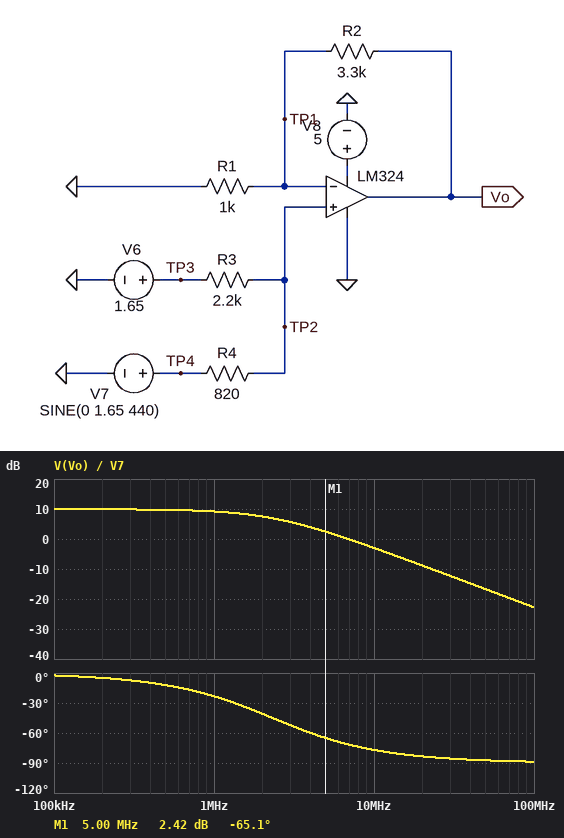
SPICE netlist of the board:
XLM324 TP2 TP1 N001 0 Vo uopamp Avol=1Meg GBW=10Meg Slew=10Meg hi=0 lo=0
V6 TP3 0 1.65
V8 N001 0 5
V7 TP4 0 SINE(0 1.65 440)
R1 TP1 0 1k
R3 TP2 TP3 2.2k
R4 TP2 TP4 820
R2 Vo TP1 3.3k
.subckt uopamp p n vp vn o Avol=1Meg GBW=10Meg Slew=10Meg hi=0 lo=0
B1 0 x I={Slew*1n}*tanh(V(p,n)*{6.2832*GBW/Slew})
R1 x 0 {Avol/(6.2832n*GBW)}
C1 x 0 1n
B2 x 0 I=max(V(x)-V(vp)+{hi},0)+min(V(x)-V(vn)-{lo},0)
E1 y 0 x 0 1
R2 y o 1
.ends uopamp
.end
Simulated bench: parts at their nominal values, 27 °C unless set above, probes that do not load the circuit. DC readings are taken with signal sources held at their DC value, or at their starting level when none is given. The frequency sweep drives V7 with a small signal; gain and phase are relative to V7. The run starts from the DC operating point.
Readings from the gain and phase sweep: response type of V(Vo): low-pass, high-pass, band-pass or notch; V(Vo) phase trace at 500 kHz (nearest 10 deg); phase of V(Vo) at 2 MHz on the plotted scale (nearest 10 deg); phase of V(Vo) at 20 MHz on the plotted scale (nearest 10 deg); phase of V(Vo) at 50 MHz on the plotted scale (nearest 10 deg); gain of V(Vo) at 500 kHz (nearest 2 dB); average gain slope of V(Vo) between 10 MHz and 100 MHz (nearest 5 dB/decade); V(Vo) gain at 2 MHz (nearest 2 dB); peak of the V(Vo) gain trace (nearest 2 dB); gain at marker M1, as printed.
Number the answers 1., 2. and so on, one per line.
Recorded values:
1. low-pass
2. -10 deg
3. -40 deg
4. -80 deg
5. -90 deg
6. 10 dB
7. -20 dB/decade
8. 8 dB
9. 10 dB
10. 2.42 dB
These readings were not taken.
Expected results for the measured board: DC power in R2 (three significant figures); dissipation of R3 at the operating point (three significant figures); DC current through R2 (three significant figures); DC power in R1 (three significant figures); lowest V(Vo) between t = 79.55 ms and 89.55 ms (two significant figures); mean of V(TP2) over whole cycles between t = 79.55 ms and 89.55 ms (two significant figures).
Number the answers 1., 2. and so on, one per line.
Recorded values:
1. 662 µW
2. 657 µW
3. 448 µA
4. 201 µW
5. -10 mV
6. 450 mV
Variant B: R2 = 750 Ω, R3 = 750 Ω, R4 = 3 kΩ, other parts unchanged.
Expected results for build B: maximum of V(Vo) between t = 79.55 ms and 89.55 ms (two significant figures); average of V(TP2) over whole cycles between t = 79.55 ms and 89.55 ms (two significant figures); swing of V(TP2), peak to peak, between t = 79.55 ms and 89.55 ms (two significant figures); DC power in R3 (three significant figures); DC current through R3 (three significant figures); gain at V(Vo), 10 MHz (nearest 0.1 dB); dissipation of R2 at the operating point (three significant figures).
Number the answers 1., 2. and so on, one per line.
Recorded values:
1. 2.9 V
2. 1.3 V
3. 660 mV
4. 145 µW
5. 440 µA
6. -15.2 dB
7. 1.31 mW
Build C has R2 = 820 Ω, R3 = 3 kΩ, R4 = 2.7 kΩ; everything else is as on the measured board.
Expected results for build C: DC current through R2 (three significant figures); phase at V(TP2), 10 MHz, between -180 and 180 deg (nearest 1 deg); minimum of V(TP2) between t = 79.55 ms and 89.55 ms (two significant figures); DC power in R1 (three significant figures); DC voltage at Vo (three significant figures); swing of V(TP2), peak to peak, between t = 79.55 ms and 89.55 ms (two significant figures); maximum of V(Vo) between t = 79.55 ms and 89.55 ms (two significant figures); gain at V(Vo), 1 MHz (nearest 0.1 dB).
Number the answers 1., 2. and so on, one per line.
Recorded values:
1. 782 µA
2. 0 deg
3. -87 mV
4. 611 µW
5. 1.42 V
6. 1.7 V
7. 3.0 V
8. -0.5 dB
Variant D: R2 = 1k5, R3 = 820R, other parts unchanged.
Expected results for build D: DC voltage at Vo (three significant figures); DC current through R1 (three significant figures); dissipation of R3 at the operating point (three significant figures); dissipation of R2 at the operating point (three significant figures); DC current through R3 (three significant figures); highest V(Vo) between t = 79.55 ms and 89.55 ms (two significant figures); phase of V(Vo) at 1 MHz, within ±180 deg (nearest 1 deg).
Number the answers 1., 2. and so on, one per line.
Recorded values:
1. 2.06 V
2. 825 µA
3. 830 µW
4. 1.02 mW
5. 1.01 mA
6. 4.1 V
7. -14 deg
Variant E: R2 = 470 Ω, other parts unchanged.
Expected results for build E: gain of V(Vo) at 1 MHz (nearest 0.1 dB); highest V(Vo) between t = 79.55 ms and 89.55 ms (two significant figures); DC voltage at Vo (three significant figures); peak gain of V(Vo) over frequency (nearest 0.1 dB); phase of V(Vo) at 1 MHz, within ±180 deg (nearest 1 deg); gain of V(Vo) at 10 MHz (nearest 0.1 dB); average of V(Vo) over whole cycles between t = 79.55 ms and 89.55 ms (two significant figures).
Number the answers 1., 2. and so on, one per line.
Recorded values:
1. 0.5 dB
2. 2.4 V
3. 659 mV
4. 0.6 dB
5. -8 deg
6. -4.4 dB
7. 930 mV
